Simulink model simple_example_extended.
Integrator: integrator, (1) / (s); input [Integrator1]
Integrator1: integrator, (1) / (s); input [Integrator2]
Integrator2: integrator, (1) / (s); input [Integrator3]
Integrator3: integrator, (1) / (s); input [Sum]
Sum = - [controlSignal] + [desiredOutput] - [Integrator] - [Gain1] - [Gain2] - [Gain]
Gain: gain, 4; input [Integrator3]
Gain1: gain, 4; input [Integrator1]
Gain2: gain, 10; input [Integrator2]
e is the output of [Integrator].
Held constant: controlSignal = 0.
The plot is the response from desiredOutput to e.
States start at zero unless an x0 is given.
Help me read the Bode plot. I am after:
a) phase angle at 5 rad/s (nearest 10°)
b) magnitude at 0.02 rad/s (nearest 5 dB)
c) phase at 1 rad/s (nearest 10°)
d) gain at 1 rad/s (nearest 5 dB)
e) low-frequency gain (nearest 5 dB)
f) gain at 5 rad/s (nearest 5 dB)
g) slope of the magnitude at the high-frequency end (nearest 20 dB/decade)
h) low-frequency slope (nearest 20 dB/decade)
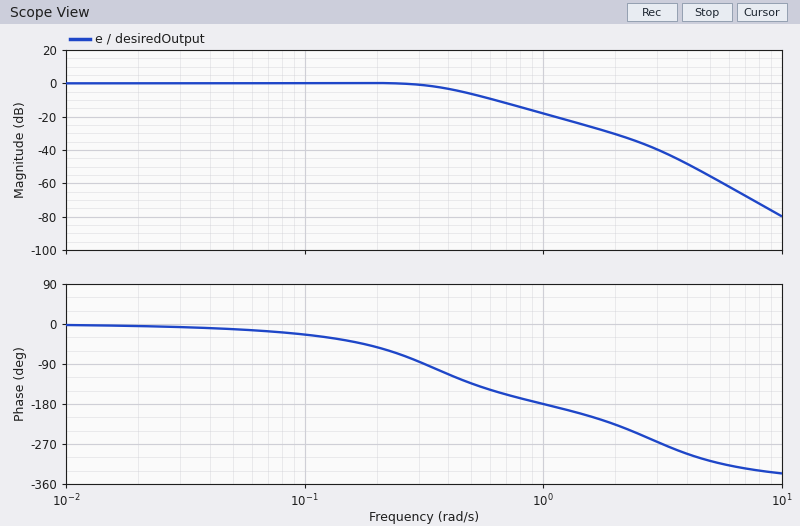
-310°
0 dB
-180°
-20 dB
0 dB
-55 dB
-80 dB/decade
0 dB/decade
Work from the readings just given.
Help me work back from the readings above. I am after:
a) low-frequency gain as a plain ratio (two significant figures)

1.0
